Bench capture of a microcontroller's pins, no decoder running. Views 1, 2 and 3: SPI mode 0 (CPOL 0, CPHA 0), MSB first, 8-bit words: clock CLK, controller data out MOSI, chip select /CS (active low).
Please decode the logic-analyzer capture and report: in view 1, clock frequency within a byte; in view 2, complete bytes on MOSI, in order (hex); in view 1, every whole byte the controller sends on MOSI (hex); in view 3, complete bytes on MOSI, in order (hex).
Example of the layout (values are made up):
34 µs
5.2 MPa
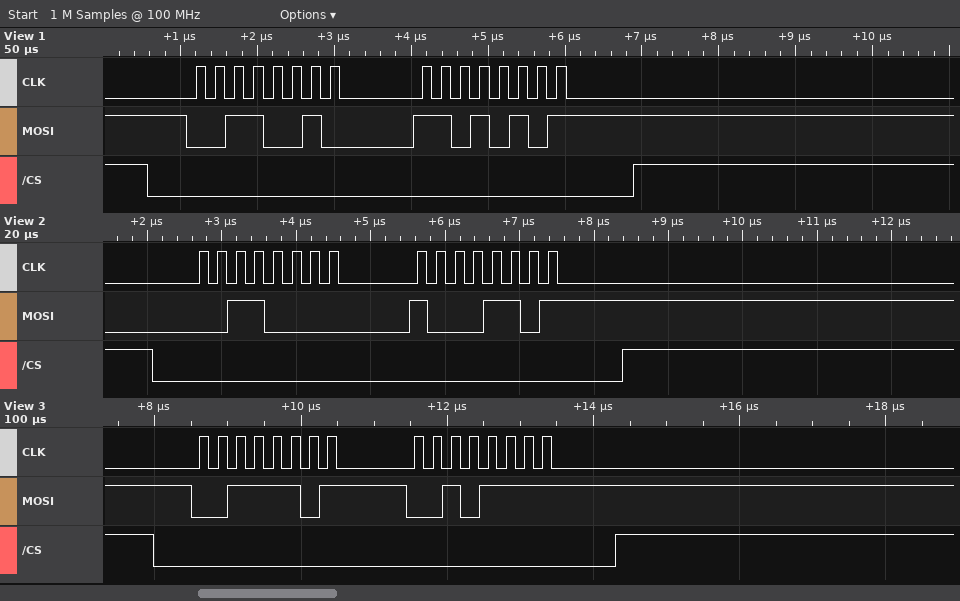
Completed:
4 MHz
30 8D
32 D5
0x3D 0x2F
